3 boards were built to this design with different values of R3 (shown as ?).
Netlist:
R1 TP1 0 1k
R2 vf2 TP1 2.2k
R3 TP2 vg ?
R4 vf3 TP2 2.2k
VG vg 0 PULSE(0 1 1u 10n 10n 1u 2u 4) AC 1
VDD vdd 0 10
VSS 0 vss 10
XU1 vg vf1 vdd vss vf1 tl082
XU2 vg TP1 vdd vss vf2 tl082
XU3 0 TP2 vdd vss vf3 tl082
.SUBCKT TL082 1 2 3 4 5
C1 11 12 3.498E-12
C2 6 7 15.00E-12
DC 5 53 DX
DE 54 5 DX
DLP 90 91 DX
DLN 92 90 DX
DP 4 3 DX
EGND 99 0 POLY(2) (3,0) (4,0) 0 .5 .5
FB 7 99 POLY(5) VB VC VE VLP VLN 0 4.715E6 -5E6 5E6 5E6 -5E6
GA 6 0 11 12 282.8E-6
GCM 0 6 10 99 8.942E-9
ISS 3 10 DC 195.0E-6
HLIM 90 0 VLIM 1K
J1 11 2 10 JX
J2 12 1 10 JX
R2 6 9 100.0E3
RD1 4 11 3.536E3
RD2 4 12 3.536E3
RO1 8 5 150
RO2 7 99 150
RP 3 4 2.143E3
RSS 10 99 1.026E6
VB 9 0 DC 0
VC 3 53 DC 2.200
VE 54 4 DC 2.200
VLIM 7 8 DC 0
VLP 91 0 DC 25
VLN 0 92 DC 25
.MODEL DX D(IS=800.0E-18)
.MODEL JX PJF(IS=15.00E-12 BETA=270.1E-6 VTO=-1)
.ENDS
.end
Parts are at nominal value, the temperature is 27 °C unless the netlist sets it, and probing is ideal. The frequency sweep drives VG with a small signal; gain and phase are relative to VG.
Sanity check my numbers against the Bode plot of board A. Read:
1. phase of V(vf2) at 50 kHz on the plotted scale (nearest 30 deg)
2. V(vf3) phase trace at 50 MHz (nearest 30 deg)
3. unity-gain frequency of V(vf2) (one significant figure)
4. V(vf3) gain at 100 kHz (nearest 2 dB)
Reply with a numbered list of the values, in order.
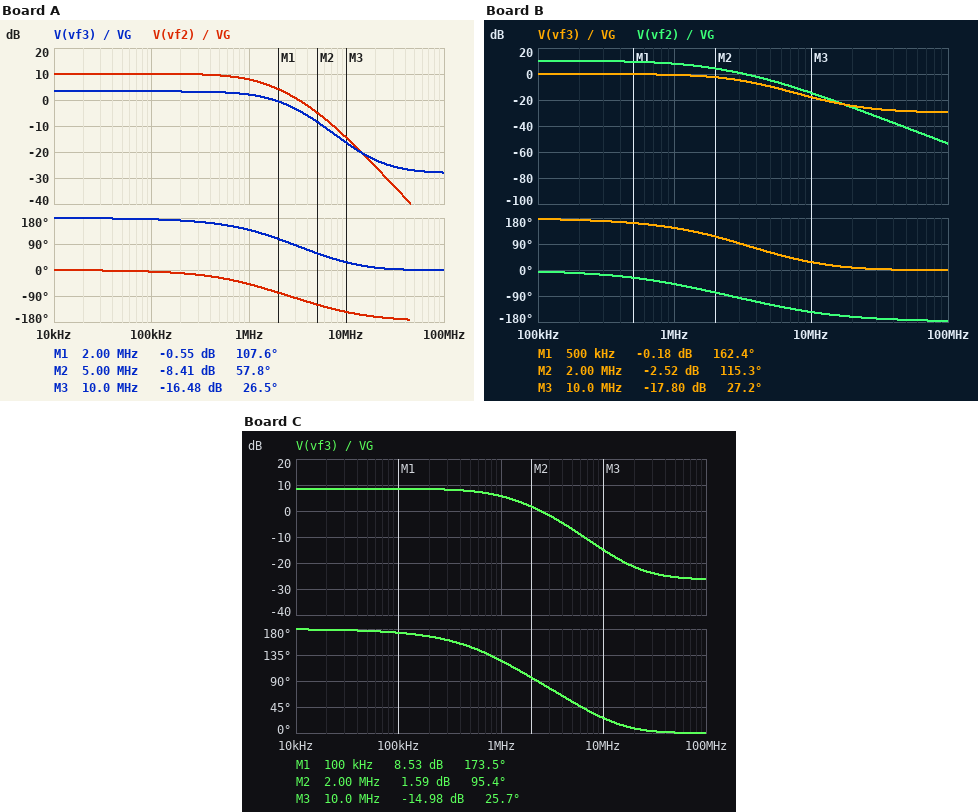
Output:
1. 0 deg
2. 0 deg
3. 3 MHz
4. 4 dB
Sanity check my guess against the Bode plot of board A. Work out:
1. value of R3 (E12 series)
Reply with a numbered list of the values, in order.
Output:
1. 1.5 kΩ
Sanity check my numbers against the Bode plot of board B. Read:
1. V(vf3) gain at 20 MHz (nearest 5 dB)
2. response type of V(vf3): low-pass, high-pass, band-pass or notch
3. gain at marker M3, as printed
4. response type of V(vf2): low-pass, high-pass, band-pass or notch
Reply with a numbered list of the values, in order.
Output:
1. -25 dB
2. low-pass
3. -17.80 dB
4. low-pass
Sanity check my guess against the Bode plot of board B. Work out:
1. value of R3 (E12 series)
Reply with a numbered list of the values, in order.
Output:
1. 2.2 kΩ
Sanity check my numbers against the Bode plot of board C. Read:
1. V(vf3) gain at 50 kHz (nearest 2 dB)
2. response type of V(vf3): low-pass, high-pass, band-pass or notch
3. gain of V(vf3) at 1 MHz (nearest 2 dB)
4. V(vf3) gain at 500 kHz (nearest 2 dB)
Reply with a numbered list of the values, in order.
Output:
1. 8 dB
2. low-pass
3. 6 dB
4. 8 dB
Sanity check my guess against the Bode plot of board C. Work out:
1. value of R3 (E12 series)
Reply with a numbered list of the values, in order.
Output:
1. 820 Ω
